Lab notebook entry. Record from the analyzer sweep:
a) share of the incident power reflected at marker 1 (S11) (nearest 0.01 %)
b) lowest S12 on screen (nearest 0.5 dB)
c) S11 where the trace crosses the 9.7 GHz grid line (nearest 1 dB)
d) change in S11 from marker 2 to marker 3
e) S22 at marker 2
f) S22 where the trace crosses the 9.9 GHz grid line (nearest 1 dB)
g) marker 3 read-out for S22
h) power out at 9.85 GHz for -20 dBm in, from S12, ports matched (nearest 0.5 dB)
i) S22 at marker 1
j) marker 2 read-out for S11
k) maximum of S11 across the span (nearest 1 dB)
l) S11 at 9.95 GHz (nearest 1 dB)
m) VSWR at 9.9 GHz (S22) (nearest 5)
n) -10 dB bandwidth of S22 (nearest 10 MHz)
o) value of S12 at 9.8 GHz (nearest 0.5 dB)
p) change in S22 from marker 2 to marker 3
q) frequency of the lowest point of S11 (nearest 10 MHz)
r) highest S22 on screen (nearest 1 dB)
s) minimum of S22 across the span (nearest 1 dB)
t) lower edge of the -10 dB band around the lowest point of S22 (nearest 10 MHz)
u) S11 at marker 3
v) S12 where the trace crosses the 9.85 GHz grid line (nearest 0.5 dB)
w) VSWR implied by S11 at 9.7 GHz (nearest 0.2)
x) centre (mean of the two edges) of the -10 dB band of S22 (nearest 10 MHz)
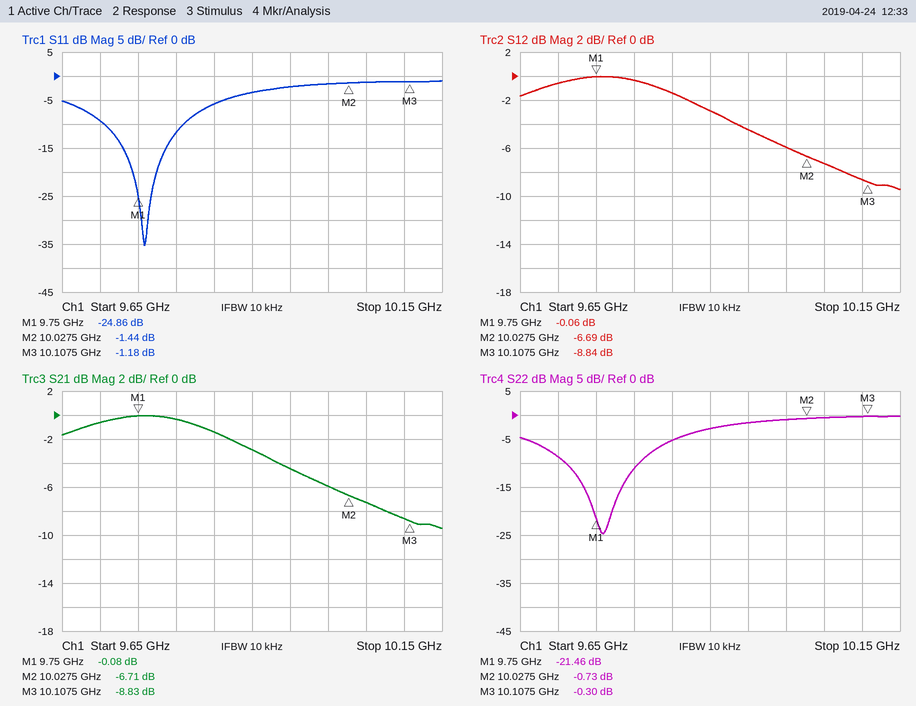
0.33 %
-9.5 dB
-9 dB
0.26 dB
-0.73 dB
-3 dB
-0.30 dB
-21.5 dBm
-21.46 dB
-1.44 dB
-1 dB
-2 dB
5
100 MHz
-0.5 dB
0.43 dB
9.76 GHz
0 dB
-25 dB
9.71 GHz
-1.18 dB
-1.5 dB
2.0
9.76 GHz
